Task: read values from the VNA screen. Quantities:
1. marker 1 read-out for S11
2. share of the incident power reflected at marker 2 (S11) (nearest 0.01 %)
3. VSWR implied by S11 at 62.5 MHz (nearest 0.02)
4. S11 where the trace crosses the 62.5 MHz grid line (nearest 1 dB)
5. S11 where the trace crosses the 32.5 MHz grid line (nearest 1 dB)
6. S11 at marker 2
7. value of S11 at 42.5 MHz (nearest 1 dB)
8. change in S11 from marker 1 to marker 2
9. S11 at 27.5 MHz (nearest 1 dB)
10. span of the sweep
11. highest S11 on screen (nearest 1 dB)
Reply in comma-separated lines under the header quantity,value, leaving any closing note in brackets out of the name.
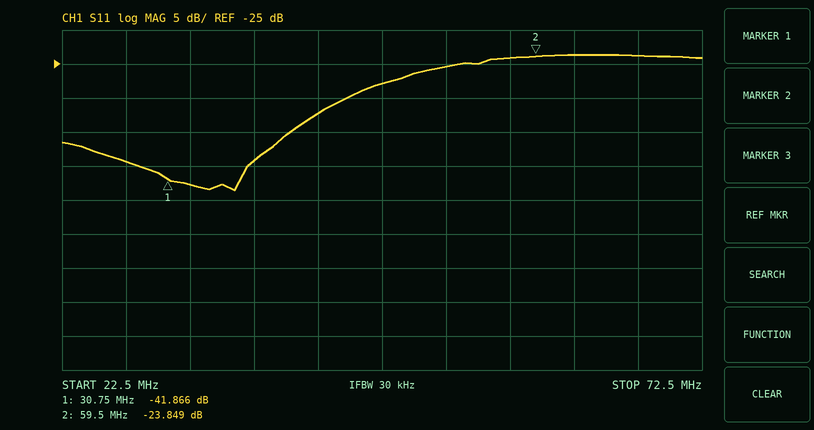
quantity,value
marker 1 read-out for S11,-41.866 dB
share of the incident power reflected at marker 2 (S11),0.41 %
VSWR implied by S11 at 62.5 MHz,1.14
S11 where the trace crosses the 62.5 MHz grid line,-24 dB
S11 where the trace crosses the 32.5 MHz grid line,-43 dB
S11 at marker 2,-23.849 dB
value of S11 at 42.5 MHz,-32 dB
change in S11 from marker 1 to marker 2,18.017 dB
S11 at 27.5 MHz,-39 dB
span of the sweep,50 MHz
highest S11 on screen,-24 dB
